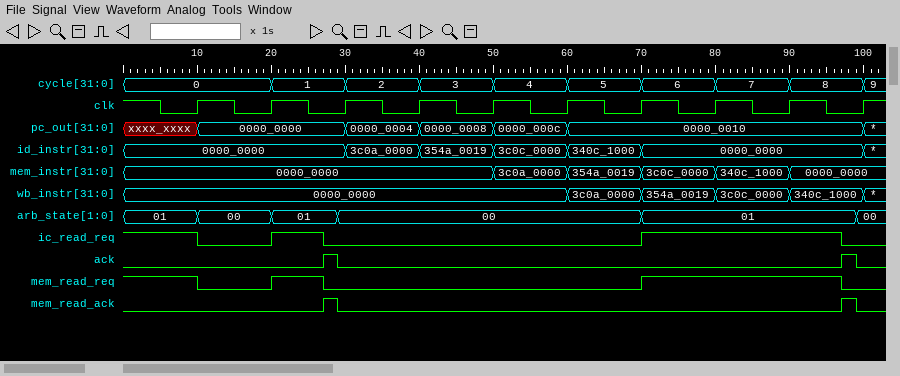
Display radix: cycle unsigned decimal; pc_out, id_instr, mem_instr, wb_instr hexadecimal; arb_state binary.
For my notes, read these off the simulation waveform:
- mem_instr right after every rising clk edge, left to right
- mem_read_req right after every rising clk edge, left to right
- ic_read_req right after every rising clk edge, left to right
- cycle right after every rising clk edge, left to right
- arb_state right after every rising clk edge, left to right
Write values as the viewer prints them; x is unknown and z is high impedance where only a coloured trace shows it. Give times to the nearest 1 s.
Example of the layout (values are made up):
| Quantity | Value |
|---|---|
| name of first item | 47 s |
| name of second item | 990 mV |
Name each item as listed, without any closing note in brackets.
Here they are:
| Quantity | Value |
|---|---|
| mem_instr right after every rising clk edge, left to right | 0000_0000, 0000_0000, 0000_0000, 0000_0000, 3c0a_0000, 354a_0019, 3c0c_0000, 340c_1000, 0000_0000, 0000_0000 |
| mem_read_req right after every rising clk edge, left to right | 0 1 0 0 0 0 1 1 1 0 |
| ic_read_req right after every rising clk edge, left to right | 0 1 0 0 0 0 1 1 1 0 |
| cycle right after every rising clk edge, left to right | 0, 1, 2, 3, 4, 5, 6, 7, 8, 9 |
| arb_state right after every rising clk edge, left to right | 00, 01, 00, 00, 00, 00, 01, 01, 01, 00 |
